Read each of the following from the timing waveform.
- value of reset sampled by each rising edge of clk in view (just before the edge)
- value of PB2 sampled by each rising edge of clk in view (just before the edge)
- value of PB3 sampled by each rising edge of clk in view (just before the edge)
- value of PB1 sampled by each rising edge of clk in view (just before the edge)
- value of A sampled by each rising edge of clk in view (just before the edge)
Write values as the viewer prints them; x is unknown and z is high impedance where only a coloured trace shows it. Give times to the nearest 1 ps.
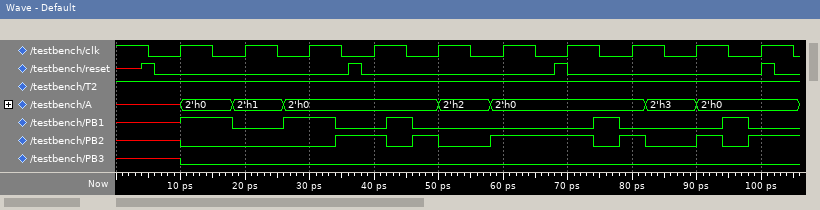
0 0 0 0 0 0 1 0 0 0
x 0 0 1 1 1 1 1 0 1
x 0 0 0 0 0 0 0 0 0
x 0 1 0 0 0 0 0 0 0
x, 2'h1, 2'h0, 2'h0, 2'h0, 2'h0, 2'h0, 2'h0, 2'h3, 2'h0
